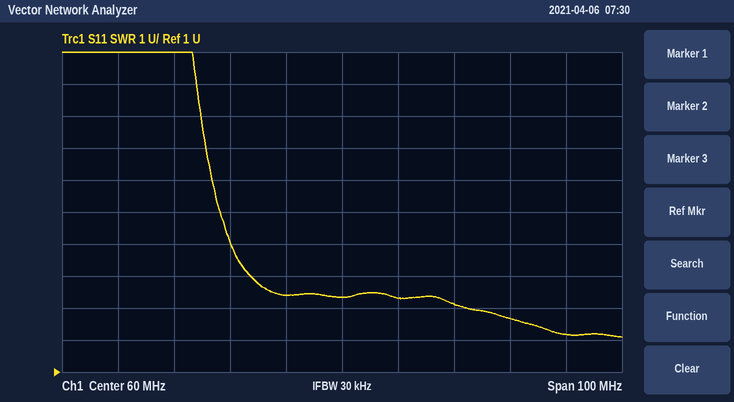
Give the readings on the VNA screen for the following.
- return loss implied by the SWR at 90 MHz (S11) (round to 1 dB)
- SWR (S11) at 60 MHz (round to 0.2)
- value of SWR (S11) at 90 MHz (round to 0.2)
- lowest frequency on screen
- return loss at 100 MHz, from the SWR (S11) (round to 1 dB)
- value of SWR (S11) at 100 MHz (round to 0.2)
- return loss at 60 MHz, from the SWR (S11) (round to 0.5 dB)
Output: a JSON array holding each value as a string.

["7 dB", "3.4", "2.6", "10 MHz", "9 dB", "2.2", "5.5 dB"]
